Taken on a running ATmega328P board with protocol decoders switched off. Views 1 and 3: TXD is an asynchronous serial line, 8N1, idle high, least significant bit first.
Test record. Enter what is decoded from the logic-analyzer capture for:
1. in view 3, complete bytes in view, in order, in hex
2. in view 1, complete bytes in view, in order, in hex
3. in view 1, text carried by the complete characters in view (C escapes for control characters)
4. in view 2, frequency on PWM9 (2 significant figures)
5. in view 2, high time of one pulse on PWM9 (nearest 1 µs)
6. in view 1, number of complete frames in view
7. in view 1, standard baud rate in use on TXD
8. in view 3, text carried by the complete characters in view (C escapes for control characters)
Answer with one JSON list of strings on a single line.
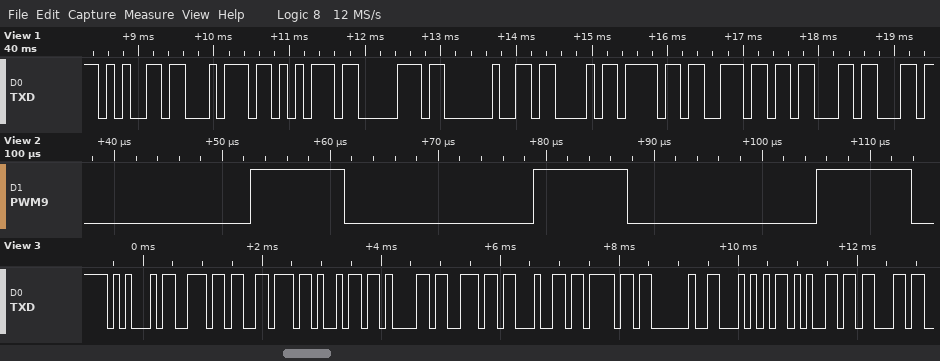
["45 6E 76 69 61 6E 64 6F 20 54 65 63", "65 74 75 70 20 43 6F 6E 63", "\"etup Conc\"", "38 kHz", "9 µs", "9", "9600 baud", "\"Enviando Tec\""]
